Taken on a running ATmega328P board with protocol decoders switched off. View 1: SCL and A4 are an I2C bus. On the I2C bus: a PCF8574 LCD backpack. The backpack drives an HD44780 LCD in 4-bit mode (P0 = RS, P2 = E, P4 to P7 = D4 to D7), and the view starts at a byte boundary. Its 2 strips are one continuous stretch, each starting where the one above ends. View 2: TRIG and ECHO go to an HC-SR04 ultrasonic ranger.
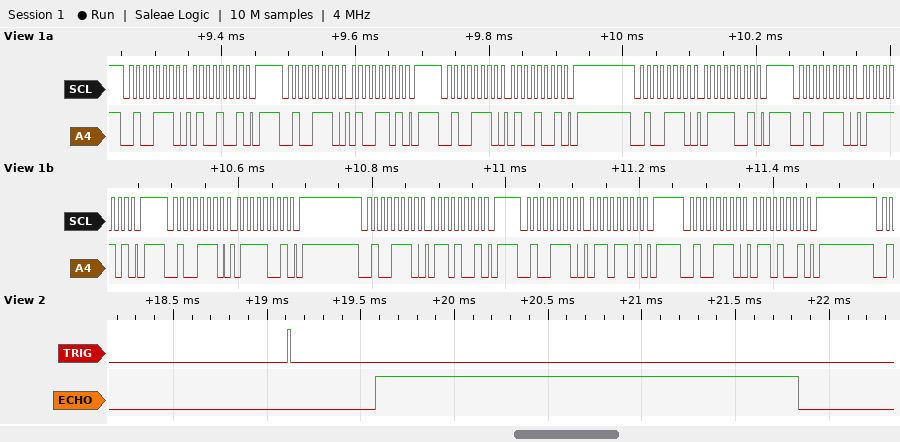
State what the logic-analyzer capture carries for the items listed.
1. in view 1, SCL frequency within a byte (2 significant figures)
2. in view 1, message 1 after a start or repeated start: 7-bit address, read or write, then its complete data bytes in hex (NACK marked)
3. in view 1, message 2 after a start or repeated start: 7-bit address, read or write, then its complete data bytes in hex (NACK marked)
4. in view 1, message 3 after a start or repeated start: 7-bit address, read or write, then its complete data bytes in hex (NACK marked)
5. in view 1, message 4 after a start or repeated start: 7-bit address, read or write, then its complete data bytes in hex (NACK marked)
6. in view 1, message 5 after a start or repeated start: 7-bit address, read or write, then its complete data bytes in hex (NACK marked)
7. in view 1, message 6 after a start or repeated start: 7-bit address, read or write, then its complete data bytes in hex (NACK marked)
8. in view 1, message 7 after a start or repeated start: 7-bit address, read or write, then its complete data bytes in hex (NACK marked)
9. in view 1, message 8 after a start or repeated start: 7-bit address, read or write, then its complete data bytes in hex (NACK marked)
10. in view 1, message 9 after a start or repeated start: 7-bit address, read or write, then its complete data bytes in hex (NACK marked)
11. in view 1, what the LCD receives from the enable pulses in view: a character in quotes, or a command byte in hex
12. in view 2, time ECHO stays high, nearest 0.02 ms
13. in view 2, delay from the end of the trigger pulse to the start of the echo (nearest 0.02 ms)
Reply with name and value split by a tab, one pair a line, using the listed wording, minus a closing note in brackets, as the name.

in view 1, SCL frequency within a byte	100 kHz
in view 1, message 1 after a start or repeated start: 7-bit address, read or write, then its complete data bytes in hex	0x27 write: 49
in view 1, message 2 after a start or repeated start: 7-bit address, read or write, then its complete data bytes in hex	0x27 write: 4D
in view 1, message 3 after a start or repeated start: 7-bit address, read or write, then its complete data bytes in hex	0x27 write: 49
in view 1, message 4 after a start or repeated start: 7-bit address, read or write, then its complete data bytes in hex	0x27 write: 79
in view 1, message 5 after a start or repeated start: 7-bit address, read or write, then its complete data bytes in hex	0x27 write: 7D
in view 1, message 6 after a start or repeated start: 7-bit address, read or write, then its complete data bytes in hex	0x27 write: 79
in view 1, message 7 after a start or repeated start: 7-bit address, read or write, then its complete data bytes in hex	0x27 write: 69
in view 1, message 8 after a start or repeated start: 7-bit address, read or write, then its complete data bytes in hex	0x27 write: 6D
in view 1, message 9 after a start or repeated start: 7-bit address, read or write, then its complete data bytes in hex	0x27 write: 69
in view 1, what the LCD receives from the enable pulses in view: a character in quotes, or a command byte in hex	'G'
in view 2, time ECHO stays high, nearest 0.02 ms	2.26 ms
in view 2, delay from the end of the trigger pulse to the start of the echo	0.46 ms
